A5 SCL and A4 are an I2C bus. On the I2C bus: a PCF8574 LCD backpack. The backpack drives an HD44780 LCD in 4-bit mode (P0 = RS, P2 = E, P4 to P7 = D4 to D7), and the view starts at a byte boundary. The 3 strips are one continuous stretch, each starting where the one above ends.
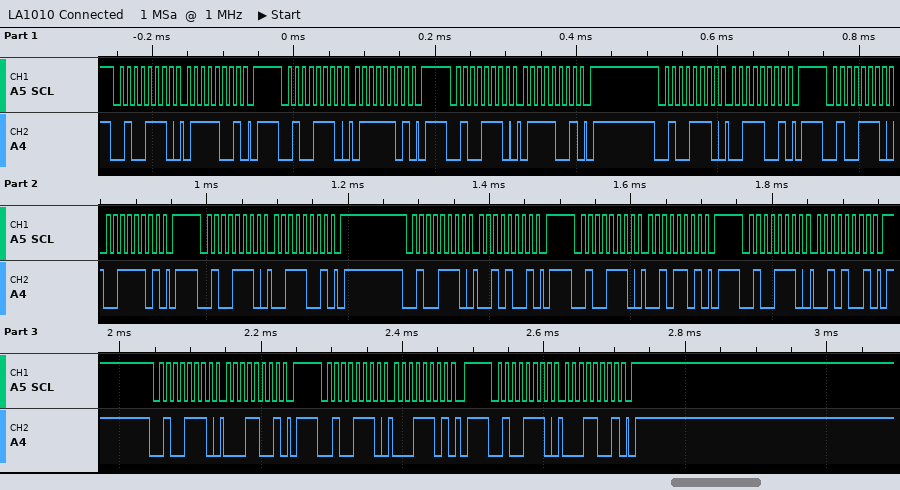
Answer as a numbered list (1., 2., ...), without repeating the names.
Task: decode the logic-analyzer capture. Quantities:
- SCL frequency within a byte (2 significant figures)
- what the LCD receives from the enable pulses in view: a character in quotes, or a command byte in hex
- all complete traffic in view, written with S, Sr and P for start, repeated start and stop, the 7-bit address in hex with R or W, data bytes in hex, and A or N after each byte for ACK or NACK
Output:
1. 100 kHz
2. 's' '!'
3. S 27W A 79 A P S 27W A 7D A P S 27W A 79 A P S 27W A 39 A P S 27W A 3D A P S 27W A 39 A P S 27W A 29 A P S 27W A 2D A P S 27W A 29 A P S 27W A 19 A P S 27W A 1D A P S 27W A 19 A P
